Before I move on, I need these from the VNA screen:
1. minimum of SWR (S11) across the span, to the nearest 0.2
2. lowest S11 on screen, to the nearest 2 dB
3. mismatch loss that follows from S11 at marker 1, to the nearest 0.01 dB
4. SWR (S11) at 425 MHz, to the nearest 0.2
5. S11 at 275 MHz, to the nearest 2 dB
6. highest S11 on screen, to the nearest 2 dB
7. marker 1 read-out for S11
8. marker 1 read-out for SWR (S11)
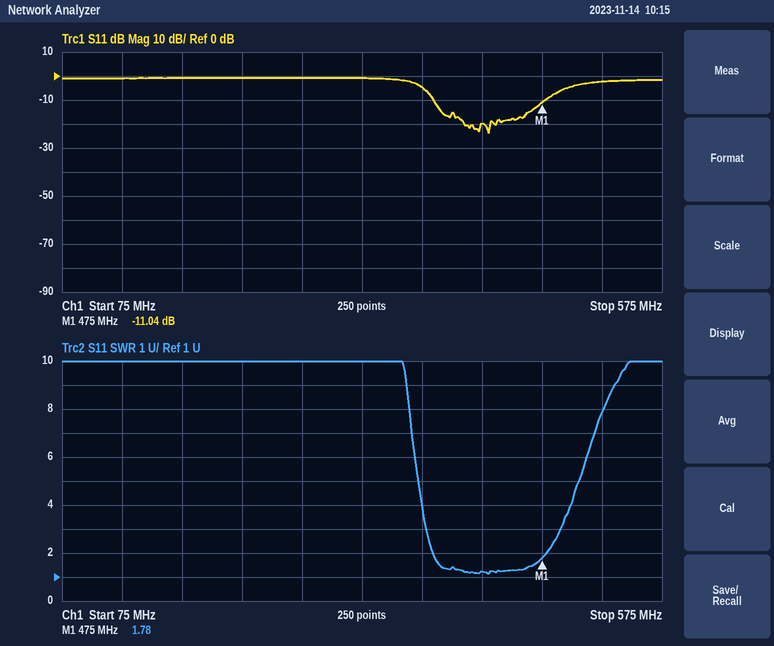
1.2
-24 dB
0.36 dB
1.2
0 dB
0 dB
-11.04 dB
1.78
